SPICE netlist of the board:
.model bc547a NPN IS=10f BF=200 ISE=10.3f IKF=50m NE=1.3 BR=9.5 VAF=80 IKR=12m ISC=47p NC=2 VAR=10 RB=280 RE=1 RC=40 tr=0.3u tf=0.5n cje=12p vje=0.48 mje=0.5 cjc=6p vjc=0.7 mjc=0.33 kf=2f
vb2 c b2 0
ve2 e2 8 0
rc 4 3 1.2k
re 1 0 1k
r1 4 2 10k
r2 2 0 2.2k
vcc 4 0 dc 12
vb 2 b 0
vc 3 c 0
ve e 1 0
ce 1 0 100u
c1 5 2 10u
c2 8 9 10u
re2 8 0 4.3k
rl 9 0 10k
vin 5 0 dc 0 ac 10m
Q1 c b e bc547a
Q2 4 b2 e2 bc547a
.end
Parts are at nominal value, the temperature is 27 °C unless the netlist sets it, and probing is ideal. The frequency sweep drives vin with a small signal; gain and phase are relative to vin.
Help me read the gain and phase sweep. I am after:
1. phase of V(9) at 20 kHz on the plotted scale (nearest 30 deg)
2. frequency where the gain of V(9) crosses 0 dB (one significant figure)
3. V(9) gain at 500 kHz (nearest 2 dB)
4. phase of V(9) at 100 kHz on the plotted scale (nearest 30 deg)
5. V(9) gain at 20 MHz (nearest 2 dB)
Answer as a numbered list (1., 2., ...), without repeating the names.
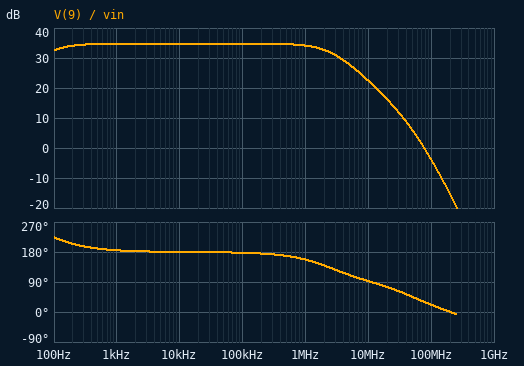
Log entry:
1. 180 deg
2. 80 MHz
3. 34 dB
4. 180 deg
5. 16 dB
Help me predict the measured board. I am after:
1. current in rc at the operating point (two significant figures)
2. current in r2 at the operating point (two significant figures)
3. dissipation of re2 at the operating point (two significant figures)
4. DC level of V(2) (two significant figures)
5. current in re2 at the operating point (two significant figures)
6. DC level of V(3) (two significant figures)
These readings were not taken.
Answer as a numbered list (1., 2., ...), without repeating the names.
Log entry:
1. 1.5 mA
2. 970 µA
3. 21 mW
4. 2.1 V
5. 2.2 mA
6. 10 V
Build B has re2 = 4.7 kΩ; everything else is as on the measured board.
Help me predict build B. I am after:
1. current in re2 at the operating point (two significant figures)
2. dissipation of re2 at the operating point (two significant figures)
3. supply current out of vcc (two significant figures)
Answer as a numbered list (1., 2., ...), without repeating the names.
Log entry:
1. 2.0 mA
2. 19 mW
3. 4.5 mA
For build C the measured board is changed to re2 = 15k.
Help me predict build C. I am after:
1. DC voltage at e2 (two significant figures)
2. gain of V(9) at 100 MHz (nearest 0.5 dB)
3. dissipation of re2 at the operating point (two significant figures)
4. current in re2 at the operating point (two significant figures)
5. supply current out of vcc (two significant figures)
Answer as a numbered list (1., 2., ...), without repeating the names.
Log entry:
1. 9.6 V
2. -3.5 dB
3. 6.1 mW
4. 640 µA
5. 3.1 mA
